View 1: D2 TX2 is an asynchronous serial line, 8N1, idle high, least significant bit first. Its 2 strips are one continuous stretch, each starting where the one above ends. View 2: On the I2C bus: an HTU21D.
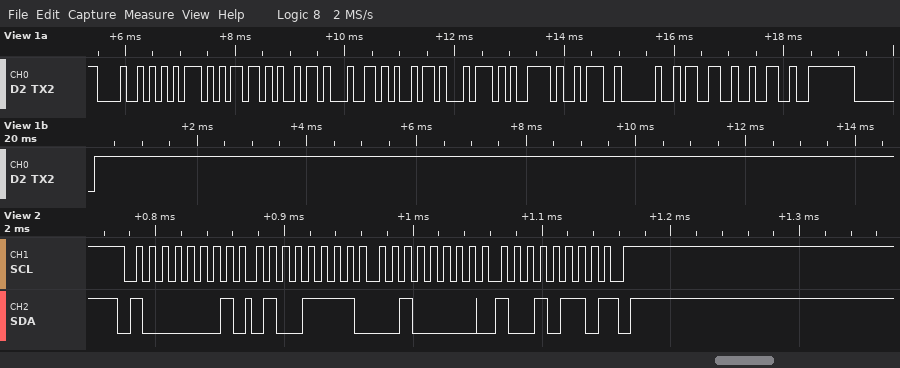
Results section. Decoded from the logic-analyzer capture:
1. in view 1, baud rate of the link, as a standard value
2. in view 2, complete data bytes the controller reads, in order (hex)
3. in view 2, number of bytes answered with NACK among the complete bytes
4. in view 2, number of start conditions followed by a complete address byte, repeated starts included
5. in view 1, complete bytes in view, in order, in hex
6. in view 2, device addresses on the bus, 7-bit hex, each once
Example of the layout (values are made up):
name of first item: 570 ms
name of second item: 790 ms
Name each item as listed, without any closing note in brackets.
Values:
in view 1, baud rate of the link, as a standard value: 9600 baud
in view 2, complete data bytes the controller reads, in order: 4F 20 96
in view 2, number of bytes answered with NACK among the complete bytes: 1
in view 2, number of start conditions followed by a complete address byte, repeated starts included: 1
in view 1, complete bytes in view, in order, in hex: 48 75 6D 69 64 69 74 79 3A 20 33 32 FE 80
in view 2, device addresses on the bus, 7-bit hex, each once: 0x40
